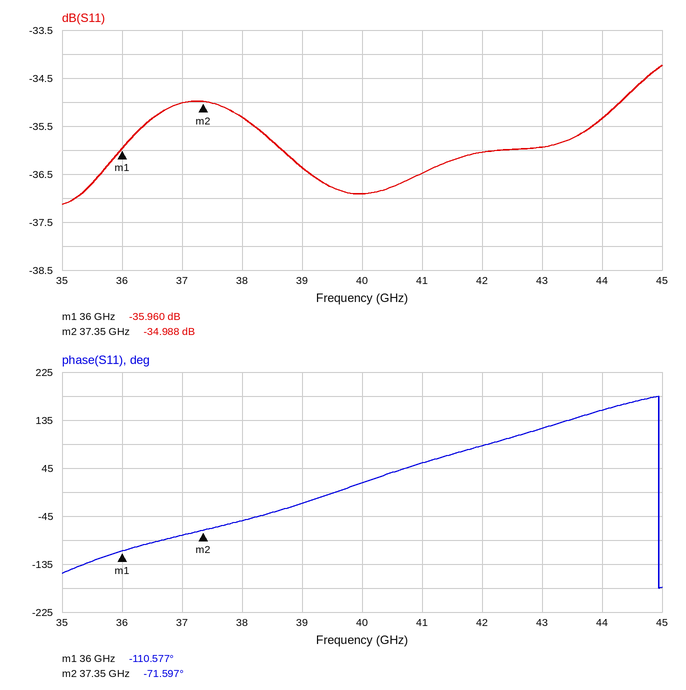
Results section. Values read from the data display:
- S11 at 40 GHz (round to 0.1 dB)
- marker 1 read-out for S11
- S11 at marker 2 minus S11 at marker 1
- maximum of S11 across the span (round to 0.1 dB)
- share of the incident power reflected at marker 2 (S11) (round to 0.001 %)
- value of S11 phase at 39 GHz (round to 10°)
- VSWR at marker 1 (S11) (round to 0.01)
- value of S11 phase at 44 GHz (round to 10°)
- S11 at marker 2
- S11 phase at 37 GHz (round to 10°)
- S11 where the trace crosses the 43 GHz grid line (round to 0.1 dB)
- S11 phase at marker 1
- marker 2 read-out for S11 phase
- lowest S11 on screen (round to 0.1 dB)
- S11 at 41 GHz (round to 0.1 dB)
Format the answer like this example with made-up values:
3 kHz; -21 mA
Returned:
-36.9 dB; -35.960 dB; 0.972 dB; -34.2 dB; 0.032 %; -20°; 1.03; 150°; -34.988 dB; -80°; -35.9 dB; -110.577°; -71.597°; -37.1 dB; -36.5 dB
